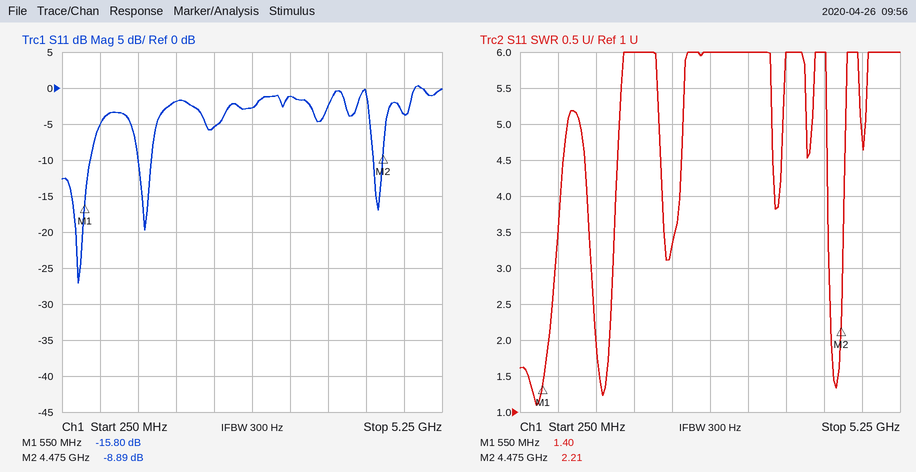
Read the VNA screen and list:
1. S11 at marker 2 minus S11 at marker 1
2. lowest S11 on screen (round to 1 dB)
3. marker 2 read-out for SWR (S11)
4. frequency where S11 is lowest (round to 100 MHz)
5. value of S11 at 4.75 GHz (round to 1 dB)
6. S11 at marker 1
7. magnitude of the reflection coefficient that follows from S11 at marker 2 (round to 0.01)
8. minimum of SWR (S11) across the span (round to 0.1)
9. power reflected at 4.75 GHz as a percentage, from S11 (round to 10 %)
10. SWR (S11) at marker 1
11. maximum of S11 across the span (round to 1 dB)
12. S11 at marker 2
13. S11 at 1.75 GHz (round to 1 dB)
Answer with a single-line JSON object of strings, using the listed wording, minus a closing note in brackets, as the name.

{"S11 at marker 2 minus S11 at marker 1": "6.91 dB", "lowest S11 on screen": "-27 dB", "marker 2 read-out for SWR": "2.21", "frequency where S11 is lowest": "500 MHz", "value of S11 at 4.75 GHz": "-4 dB", "S11 at marker 1": "-15.80 dB", "magnitude of the reflection coefficient that follows from S11 at marker 2": "0.36", "minimum of SWR (S11) across the span": "1.1", "power reflected at 4.75 GHz as a percentage, from S11": "40 %", "SWR (S11) at marker 1": "1.40", "maximum of S11 across the span": "0 dB", "S11 at marker 2": "-8.89 dB", "S11 at 1.75 GHz": "-2 dB"}
